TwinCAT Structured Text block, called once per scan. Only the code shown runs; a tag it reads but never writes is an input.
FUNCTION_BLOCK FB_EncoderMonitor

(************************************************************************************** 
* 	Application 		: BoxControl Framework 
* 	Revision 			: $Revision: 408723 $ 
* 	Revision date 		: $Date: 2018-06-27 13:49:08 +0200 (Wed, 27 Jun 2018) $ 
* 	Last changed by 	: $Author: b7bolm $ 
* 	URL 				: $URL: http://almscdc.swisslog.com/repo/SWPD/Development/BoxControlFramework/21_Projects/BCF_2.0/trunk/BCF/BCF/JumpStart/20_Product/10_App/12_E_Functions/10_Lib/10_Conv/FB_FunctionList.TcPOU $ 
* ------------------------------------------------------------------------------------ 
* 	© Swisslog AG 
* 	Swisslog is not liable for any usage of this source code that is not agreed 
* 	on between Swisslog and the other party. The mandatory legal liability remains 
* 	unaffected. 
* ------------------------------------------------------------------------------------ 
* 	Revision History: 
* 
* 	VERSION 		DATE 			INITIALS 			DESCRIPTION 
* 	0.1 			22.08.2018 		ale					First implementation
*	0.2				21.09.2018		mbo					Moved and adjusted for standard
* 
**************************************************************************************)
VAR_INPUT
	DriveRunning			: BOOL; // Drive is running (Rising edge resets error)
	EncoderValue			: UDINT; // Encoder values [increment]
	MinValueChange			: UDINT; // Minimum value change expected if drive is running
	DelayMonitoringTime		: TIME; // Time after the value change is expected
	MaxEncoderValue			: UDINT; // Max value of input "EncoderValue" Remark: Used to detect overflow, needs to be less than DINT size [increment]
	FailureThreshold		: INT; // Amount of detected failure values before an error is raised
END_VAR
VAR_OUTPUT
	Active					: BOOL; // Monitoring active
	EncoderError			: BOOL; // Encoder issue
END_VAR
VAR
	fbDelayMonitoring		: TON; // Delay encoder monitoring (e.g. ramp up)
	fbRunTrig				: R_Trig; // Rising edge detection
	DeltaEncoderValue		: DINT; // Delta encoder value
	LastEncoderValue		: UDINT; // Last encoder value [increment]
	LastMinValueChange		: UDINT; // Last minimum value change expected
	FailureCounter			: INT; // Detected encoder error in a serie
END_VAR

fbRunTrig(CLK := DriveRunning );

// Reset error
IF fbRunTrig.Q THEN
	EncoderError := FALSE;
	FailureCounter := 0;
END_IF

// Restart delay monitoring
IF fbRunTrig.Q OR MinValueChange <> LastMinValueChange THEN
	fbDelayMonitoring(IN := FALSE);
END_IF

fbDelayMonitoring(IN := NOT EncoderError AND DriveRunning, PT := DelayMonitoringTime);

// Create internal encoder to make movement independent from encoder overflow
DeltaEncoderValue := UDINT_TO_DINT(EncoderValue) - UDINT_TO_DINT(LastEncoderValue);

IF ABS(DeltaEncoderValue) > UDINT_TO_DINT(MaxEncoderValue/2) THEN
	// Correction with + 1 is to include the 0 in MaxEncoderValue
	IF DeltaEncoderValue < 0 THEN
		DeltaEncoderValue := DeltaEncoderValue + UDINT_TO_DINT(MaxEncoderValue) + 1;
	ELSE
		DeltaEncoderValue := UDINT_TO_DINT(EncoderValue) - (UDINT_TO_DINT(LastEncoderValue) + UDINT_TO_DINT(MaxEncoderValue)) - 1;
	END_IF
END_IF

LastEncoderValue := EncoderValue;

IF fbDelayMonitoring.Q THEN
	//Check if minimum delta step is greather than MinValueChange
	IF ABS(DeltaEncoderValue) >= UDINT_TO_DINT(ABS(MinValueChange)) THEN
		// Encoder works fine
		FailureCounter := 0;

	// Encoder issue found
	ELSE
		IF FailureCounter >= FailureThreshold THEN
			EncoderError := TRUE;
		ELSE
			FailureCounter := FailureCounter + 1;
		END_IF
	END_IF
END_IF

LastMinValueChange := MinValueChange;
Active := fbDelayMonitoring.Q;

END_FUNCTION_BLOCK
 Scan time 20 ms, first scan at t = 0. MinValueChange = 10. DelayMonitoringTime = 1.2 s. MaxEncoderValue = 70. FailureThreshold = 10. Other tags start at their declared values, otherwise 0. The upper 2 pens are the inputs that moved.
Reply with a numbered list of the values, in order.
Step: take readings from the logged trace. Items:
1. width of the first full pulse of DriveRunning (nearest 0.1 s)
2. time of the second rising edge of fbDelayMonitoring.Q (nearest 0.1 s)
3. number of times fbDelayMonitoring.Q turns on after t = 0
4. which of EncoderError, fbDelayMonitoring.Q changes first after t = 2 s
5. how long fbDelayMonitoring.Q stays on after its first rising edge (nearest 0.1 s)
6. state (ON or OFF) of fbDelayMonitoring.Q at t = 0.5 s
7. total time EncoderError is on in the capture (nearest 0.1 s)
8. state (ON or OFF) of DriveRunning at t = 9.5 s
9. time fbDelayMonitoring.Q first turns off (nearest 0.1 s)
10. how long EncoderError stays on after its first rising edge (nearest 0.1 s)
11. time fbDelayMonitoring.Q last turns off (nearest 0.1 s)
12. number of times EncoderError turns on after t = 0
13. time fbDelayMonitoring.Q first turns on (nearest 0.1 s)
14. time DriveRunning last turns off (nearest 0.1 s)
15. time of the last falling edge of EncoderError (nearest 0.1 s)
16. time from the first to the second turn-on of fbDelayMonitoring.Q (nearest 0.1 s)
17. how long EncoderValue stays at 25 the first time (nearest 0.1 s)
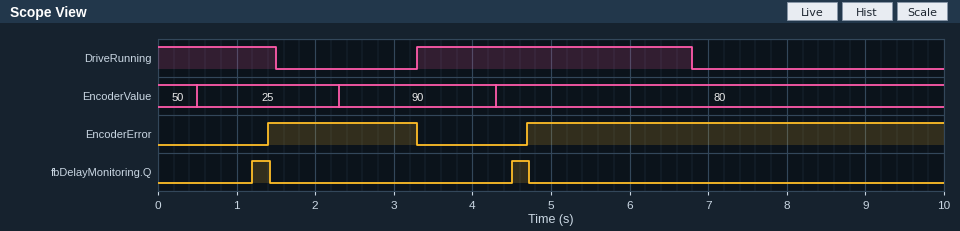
1. 3.5 s
2. 4.5 s
3. 2
4. EncoderError
5. 0.2 s
6. OFF
7. 7.2 s
8. OFF
9. 1.4 s
10. 1.9 s
11. 4.7 s
12. 2
13. 1.2 s
14. 6.8 s
15. 3.3 s
16. 3.3 s
17. 1.8 s
